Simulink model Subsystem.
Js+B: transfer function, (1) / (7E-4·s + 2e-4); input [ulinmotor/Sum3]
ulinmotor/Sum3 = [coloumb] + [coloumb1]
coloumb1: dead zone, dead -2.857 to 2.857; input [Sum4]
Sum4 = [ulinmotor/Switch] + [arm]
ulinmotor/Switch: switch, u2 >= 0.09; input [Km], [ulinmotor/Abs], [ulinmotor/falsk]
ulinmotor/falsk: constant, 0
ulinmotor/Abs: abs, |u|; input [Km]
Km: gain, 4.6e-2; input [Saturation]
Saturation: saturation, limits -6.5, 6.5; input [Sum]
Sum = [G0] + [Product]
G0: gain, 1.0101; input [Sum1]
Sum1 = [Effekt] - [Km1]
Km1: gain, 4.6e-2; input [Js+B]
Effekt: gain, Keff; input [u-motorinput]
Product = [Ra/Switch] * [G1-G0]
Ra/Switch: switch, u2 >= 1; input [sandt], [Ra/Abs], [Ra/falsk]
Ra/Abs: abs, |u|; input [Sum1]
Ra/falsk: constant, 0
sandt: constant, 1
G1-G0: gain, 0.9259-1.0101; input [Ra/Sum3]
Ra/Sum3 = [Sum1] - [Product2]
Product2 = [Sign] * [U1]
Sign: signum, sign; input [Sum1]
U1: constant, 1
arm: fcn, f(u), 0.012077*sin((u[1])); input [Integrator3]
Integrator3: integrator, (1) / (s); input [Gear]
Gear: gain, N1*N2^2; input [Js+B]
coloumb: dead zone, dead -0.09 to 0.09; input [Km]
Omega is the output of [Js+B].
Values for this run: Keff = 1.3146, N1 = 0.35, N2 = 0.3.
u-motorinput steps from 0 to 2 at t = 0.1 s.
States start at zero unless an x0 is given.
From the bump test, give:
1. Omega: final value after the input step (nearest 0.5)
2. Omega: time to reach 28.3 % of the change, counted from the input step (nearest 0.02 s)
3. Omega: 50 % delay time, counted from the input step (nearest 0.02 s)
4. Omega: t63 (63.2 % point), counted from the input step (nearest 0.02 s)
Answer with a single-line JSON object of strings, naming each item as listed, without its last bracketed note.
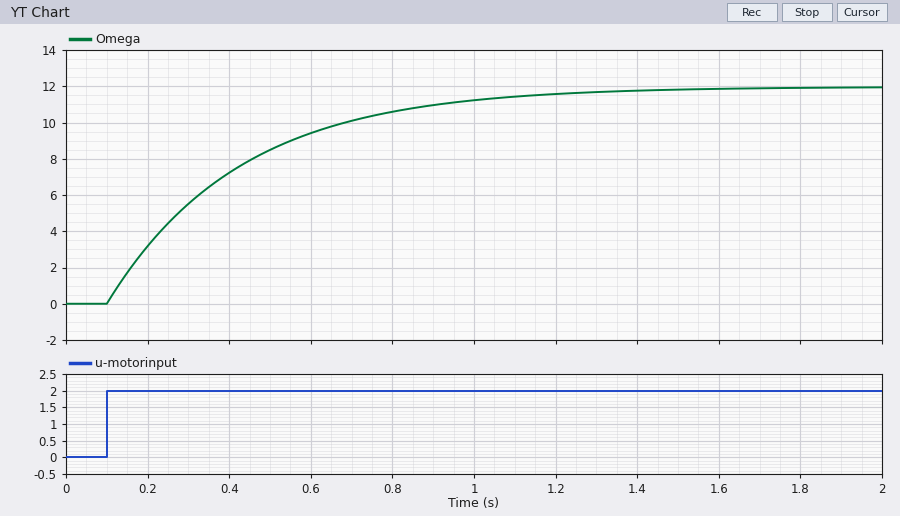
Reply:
{"Omega: final value after the input step": "12.0", "Omega: time to reach 28.3 % of the change, counted from the input step": "0.10 s", "Omega: 50 % delay time, counted from the input step": "0.22 s", "Omega: t63 (63.2 % point), counted from the input step": "0.32 s"}
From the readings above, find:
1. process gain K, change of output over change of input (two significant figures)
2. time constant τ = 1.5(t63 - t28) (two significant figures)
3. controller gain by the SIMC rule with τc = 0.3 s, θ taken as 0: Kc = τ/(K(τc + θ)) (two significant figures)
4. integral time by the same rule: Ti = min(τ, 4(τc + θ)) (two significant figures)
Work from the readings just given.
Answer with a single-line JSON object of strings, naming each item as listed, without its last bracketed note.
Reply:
{"process gain K, change of output over change of input": "6.0", "time constant τ = 1.5(t63 - t28)": "0.33 s", "controller gain by the SIMC rule with τc = 0.3 s, θ taken as 0: Kc = τ/(K(τc + θ))": "0.18", "integral time by the same rule: Ti = min(τ, 4(τc + θ))": "0.33 s"}
